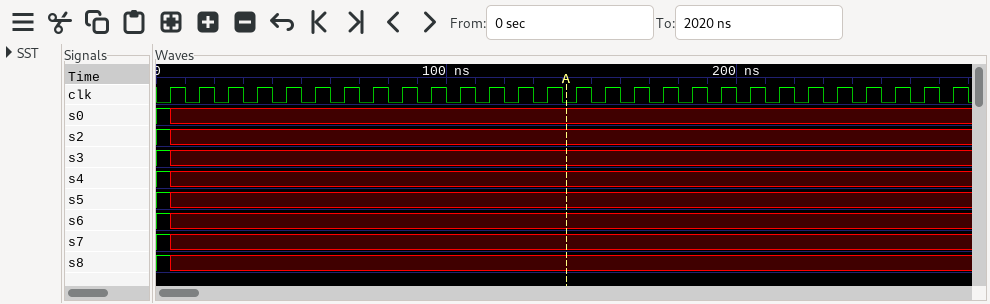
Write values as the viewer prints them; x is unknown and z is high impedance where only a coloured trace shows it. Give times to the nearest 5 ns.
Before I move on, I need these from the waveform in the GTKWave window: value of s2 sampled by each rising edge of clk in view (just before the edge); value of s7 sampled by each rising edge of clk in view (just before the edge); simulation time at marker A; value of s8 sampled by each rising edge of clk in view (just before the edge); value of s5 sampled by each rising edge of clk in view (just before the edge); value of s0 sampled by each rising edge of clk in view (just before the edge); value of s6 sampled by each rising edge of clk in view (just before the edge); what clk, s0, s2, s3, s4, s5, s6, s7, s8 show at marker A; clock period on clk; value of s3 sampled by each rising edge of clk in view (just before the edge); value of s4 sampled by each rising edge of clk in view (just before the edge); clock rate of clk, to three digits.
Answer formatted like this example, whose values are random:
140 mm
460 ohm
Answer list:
1 x x x x x x x x x x x x x x x x x x x x x x x x x x x
1 x x x x x x x x x x x x x x x x x x x x x x x x x x x
140 ns
1 x x x x x x x x x x x x x x x x x x x x x x x x x x x
1 x x x x x x x x x x x x x x x x x x x x x x x x x x x
1 x x x x x x x x x x x x x x x x x x x x x x x x x x x
1 x x x x x x x x x x x x x x x x x x x x x x x x x x x
clk=0, s0=x, s2=x, s3=x, s4=x, s5=x, s6=x, s7=x, s8=x
10 ns
1 x x x x x x x x x x x x x x x x x x x x x x x x x x x
1 x x x x x x x x x x x x x x x x x x x x x x x x x x x
100 MHz
